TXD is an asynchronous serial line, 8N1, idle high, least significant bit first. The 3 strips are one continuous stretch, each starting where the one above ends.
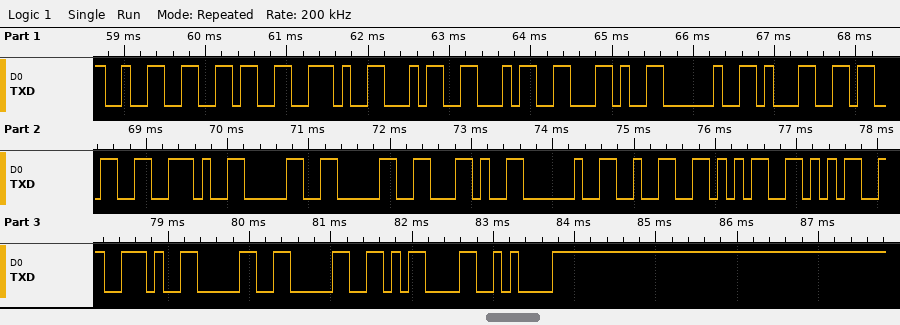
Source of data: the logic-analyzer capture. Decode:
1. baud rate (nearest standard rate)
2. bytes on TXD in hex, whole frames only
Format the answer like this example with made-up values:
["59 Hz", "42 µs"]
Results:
["9600 baud", "0x32 0x36 0x2E 0x34 0x34 0x2C 0x20 0x31 0x33 0x2E 0x30 0x30 0x2C 0x20 0x32 0x35 0x35 0x2E 0x30 0x30 0x0D 0x0A"]
